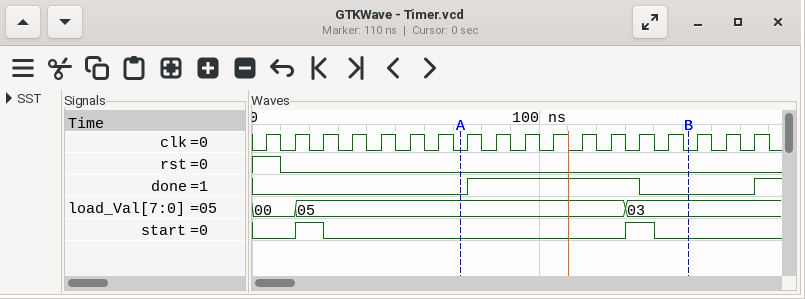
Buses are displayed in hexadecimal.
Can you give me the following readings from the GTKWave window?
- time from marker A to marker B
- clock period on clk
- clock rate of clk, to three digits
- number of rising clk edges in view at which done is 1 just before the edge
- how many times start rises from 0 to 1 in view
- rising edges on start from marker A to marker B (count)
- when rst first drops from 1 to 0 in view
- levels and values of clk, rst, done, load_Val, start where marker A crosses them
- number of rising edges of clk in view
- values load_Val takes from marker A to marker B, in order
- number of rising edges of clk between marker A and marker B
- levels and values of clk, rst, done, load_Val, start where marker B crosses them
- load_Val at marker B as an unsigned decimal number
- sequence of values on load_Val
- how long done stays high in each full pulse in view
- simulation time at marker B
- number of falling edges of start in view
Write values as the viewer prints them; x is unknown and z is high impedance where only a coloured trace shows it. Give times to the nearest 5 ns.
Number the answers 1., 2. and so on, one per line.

1. 80 ns
2. 10 ns
3. 100 MHz
4. 6
5. 2
6. 1
7. 10 ns
8. clk=0, rst=0, done=0, load_Val=05, start=0
9. 18
10. 05, 03
11. 8
12. clk=0, rst=0, done=0, load_Val=03, start=0
13. 3
14. 00, 05, 03
15. 60 ns
16. 150 ns
17. 2
